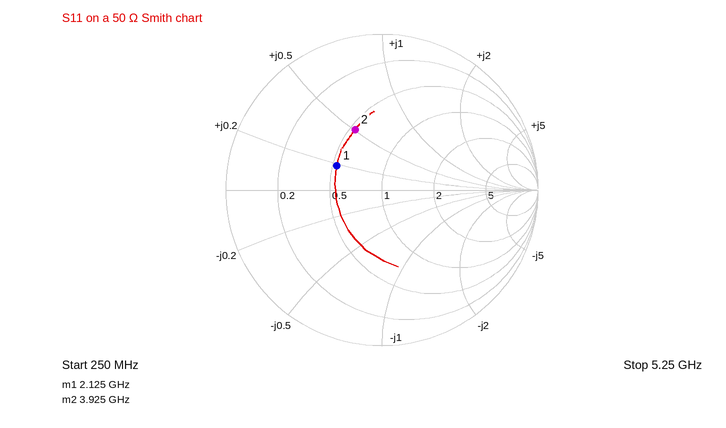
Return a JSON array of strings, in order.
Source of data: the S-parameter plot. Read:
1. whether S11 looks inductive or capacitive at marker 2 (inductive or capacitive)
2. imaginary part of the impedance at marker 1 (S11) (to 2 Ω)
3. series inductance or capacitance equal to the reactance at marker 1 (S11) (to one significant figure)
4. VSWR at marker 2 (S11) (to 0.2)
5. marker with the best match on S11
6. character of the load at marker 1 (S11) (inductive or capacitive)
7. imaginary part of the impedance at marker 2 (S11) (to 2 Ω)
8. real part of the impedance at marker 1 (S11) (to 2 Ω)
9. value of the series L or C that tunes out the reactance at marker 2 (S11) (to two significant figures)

["inductive", "+10 Ω", "700 pH", "2.4", "marker 1", "inductive", "+26 Ω", "26 Ω", "1.6 pF"]
